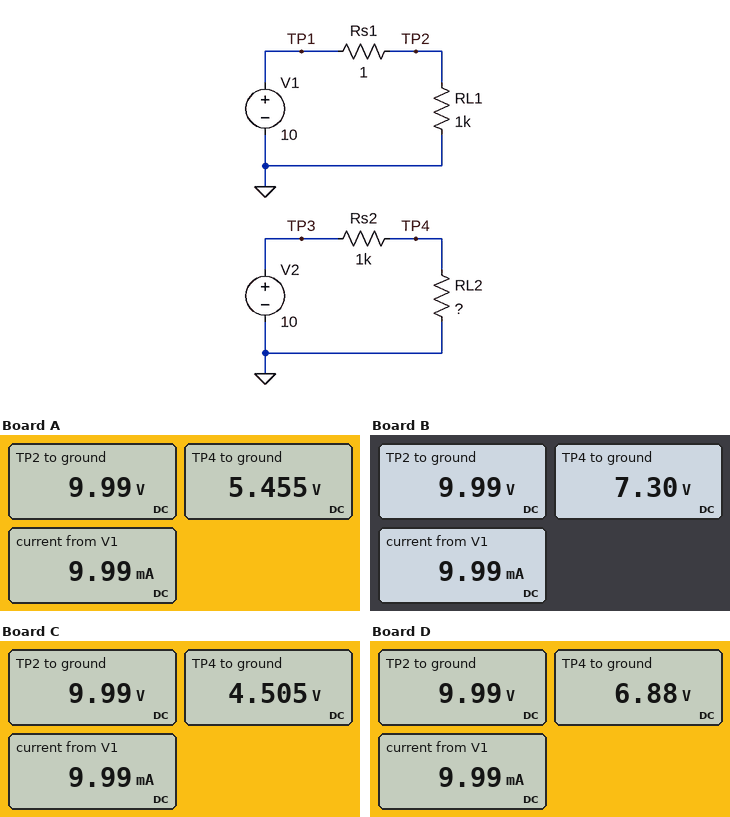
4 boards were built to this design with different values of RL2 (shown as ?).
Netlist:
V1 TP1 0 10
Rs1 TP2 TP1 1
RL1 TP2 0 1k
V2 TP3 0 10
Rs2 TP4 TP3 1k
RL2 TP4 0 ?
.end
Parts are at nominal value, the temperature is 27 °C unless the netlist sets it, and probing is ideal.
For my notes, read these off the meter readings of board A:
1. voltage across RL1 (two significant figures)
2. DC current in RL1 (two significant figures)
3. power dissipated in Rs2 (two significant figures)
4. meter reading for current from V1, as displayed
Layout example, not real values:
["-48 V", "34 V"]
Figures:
["10 V", "10 mA", "21 mW", "9.99 mA"]
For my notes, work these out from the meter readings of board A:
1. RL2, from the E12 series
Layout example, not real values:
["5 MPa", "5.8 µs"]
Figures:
["1.2 kΩ"]
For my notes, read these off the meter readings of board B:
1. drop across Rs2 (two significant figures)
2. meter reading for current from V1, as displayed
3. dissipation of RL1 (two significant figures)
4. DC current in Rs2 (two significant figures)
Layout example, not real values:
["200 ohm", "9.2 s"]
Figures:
["2.7 V", "9.99 mA", "100 mW", "2.7 mA"]
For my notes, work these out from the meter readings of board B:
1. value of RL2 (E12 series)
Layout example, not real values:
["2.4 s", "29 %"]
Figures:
["2.7 kΩ"]
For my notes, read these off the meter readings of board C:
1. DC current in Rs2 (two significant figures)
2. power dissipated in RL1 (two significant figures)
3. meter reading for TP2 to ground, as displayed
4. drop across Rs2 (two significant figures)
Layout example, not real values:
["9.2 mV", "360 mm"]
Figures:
["5.5 mA", "100 mW", "9.99 V", "5.5 V"]
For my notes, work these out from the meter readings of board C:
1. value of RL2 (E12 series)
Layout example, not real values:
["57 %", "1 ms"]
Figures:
["820 Ω"]
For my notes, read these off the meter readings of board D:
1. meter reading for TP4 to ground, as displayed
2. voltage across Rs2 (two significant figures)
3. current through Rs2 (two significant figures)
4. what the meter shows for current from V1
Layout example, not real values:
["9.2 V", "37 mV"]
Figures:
["6.88 V", "3.1 V", "3.1 mA", "9.99 mA"]
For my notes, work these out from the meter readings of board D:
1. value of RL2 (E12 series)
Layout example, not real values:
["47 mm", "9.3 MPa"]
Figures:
["2.2 kΩ"]
